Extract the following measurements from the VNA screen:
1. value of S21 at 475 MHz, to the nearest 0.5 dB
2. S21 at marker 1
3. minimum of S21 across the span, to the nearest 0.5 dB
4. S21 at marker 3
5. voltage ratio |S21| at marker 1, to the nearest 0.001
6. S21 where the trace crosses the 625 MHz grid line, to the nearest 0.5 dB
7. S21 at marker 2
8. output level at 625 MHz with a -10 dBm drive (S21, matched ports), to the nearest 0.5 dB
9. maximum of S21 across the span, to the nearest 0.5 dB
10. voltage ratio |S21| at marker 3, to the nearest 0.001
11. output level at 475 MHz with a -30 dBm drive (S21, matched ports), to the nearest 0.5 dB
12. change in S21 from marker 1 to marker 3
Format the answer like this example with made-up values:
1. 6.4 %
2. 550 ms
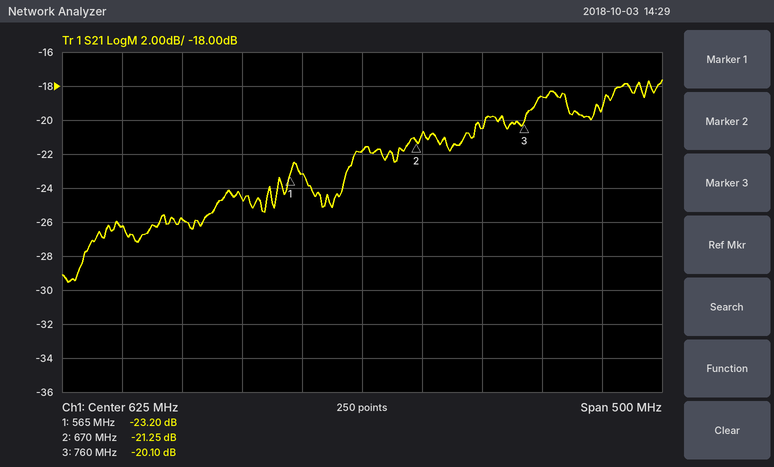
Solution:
1. -26.0 dB
2. -23.20 dB
3. -29.5 dB
4. -20.10 dB
5. 0.069
6. -22.0 dB
7. -21.25 dB
8. -32.0 dBm
9. -17.5 dB
10. 0.099
11. -56.0 dBm
12. 3.10 dB
